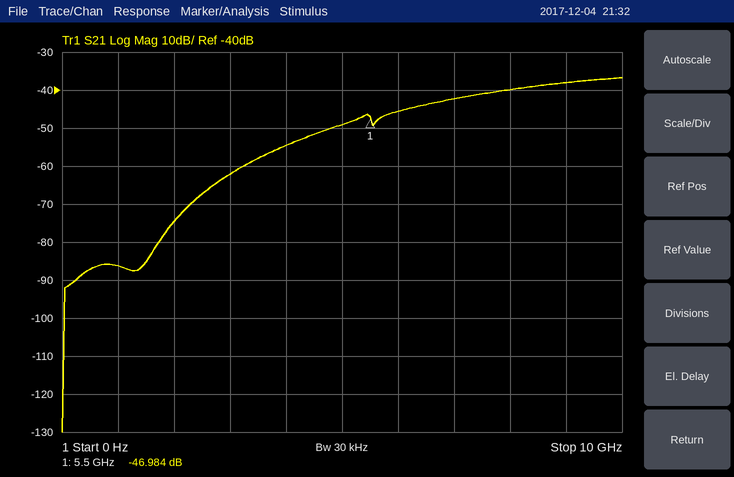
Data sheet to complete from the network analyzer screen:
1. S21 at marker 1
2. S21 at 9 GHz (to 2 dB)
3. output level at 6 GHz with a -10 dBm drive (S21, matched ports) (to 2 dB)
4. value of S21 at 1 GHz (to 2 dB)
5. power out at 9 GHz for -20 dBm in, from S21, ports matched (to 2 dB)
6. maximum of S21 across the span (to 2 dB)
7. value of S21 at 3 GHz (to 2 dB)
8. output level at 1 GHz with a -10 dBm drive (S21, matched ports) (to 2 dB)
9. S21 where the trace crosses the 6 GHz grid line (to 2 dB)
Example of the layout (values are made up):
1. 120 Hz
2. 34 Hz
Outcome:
1. -46.984 dB
2. -38 dB
3. -56 dBm
4. -86 dB
5. -58 dBm
6. -36 dB
7. -62 dB
8. -96 dBm
9. -46 dB
